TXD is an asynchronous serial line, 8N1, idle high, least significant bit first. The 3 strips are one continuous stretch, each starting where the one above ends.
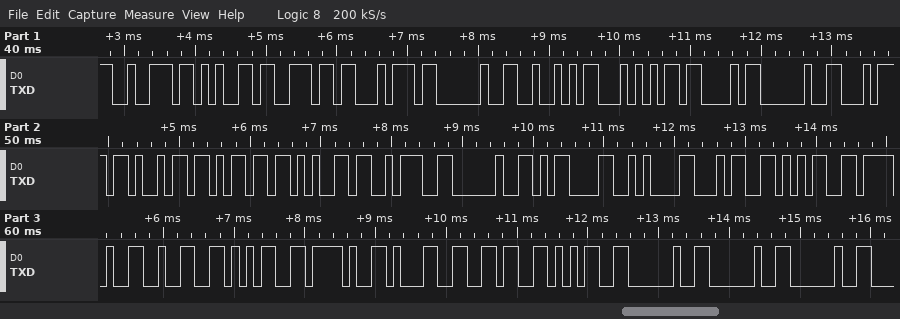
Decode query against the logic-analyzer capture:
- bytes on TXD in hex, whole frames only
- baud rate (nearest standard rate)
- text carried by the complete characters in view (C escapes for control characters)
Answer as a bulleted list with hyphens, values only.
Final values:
- 72 65 6E 74 20 52 54 43 20 74 69 6D 65 3A 20 0D 0A 34 35 2F 32 35 2F 31 36 35 20 20 20
- 9600 baud
- "rent RTC time: \r\n45/25/165   "
